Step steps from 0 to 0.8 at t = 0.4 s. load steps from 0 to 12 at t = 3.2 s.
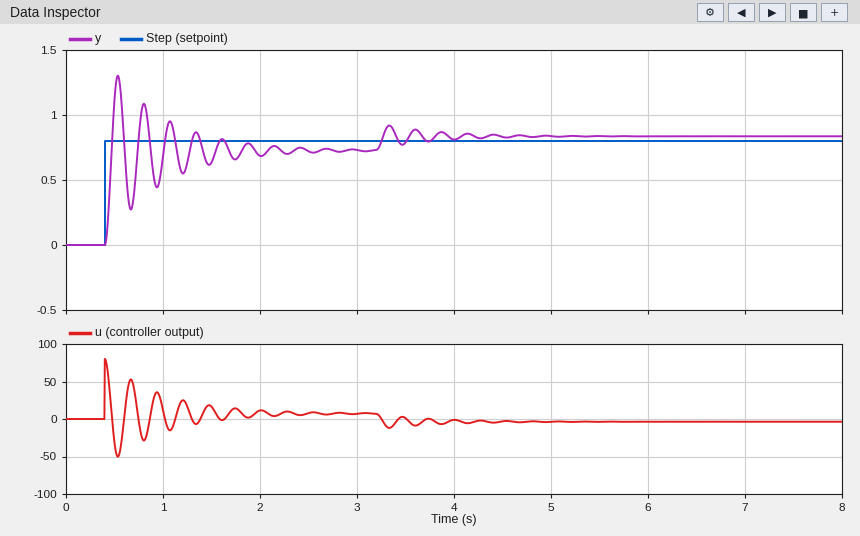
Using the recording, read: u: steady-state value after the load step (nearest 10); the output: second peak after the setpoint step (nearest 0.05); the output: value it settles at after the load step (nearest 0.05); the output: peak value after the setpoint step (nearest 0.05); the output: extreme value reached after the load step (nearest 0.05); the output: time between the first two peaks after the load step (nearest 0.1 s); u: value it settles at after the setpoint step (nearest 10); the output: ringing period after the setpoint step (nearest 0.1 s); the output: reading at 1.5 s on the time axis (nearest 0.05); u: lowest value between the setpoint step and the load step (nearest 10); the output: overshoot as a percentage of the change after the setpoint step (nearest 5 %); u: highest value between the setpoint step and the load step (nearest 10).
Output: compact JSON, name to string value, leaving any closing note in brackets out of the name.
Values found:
{"u: steady-state value after the load step": "0", "the output: second peak after the setpoint step": "1.10", "the output: value it settles at after the load step": "0.85", "the output: peak value after the setpoint step": "1.30", "the output: extreme value reached after the load step": "0.90", "the output: time between the first two peaks after the load step": "0.3 s", "u: value it settles at after the setpoint step": "10", "the output: ringing period after the setpoint step": "0.3 s", "the output: reading at 1.5 s on the time axis": "0.65", "u: lowest value between the setpoint step and the load step": "-50", "the output: overshoot as a percentage of the change after the setpoint step": "80 %", "u: highest value between the setpoint step and the load step": "80"}
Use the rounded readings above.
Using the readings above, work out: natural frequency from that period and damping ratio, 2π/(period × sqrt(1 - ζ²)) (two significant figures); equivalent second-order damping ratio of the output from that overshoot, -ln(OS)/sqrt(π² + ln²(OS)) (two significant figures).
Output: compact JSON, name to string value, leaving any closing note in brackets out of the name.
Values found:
{"natural frequency from that period and damping ratio, 2π/(period × sqrt(1 - ζ²))": "21 rad/s", "equivalent second-order damping ratio of the output from that overshoot, -ln(OS)/sqrt(π² + ln²(OS))": "0.071"}
